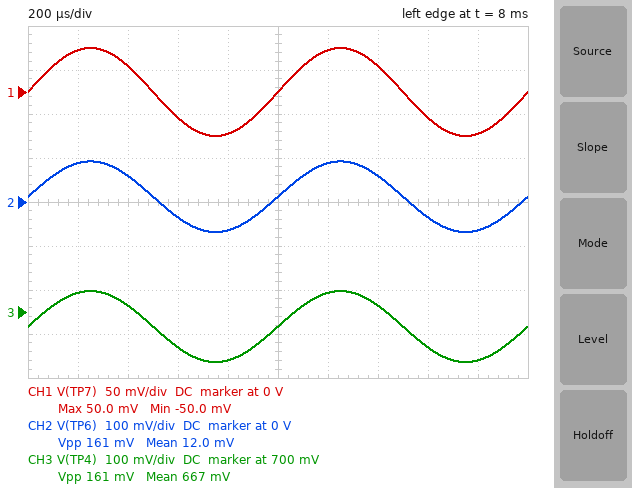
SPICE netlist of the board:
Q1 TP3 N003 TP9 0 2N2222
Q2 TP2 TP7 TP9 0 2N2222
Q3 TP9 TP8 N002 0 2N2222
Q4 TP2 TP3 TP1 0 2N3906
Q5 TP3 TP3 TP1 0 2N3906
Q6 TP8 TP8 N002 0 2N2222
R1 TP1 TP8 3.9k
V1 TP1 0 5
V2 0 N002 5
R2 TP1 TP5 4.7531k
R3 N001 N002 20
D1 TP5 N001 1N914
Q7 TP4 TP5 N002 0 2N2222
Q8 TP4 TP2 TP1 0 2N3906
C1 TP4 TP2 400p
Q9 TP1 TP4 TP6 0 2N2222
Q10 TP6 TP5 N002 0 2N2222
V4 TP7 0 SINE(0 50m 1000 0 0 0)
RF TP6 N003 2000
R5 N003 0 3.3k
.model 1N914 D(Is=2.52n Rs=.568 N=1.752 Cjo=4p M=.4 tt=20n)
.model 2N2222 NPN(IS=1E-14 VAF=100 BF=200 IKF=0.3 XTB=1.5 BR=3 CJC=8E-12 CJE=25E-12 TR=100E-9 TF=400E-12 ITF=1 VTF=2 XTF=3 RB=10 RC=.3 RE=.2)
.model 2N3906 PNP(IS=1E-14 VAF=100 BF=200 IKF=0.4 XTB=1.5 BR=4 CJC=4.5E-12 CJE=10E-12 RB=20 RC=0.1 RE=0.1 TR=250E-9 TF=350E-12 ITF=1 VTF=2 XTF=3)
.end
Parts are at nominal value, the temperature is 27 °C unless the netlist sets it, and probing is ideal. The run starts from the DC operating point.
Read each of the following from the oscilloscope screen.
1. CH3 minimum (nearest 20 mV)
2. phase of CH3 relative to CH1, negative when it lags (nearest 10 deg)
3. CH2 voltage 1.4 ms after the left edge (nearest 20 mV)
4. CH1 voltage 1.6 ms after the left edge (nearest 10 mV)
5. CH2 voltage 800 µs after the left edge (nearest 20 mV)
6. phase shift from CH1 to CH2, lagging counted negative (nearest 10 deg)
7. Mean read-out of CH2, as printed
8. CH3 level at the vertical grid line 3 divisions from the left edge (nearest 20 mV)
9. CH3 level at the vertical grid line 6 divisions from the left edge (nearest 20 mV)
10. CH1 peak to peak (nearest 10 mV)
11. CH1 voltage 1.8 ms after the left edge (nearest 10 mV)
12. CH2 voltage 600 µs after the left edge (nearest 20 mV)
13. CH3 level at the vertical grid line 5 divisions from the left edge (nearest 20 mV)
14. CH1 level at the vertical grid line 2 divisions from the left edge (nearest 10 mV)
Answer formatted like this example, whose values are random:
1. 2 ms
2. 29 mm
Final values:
1. 580 mV
2. 0 deg
3. 60 mV
4. -30 mV
5. -60 mV
6. 0 deg
7. 12.0 mV
8. 620 mV
9. 740 mV
10. 100 mV
11. -50 mV
12. -40 mV
13. 660 mV
14. 30 mV
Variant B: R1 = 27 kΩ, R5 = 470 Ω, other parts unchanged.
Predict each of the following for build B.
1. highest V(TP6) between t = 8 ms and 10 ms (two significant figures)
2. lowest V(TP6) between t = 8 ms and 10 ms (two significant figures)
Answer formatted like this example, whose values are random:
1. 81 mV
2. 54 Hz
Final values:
1. 260 mV
2. -260 mV
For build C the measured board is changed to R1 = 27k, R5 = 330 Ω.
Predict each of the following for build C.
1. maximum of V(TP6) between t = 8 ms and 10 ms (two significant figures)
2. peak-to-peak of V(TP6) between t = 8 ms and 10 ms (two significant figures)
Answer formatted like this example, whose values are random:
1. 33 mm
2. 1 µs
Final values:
1. 350 mV
2. 710 mV
